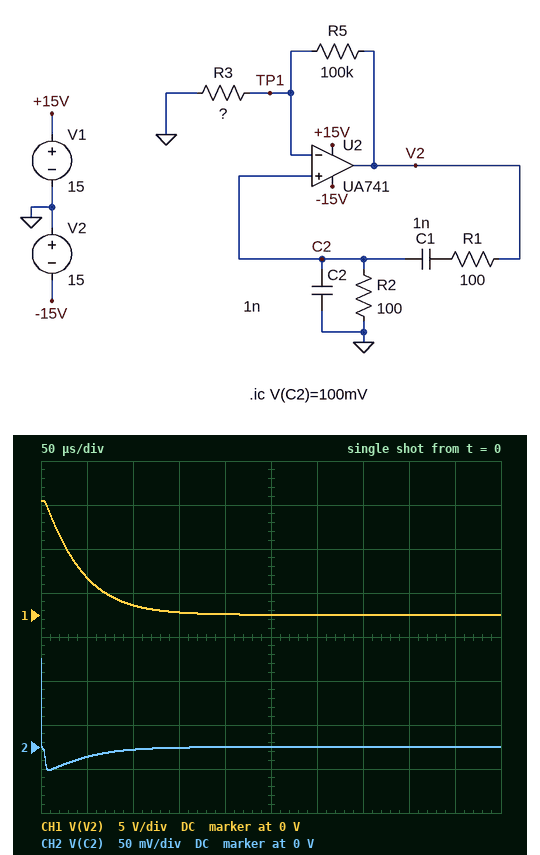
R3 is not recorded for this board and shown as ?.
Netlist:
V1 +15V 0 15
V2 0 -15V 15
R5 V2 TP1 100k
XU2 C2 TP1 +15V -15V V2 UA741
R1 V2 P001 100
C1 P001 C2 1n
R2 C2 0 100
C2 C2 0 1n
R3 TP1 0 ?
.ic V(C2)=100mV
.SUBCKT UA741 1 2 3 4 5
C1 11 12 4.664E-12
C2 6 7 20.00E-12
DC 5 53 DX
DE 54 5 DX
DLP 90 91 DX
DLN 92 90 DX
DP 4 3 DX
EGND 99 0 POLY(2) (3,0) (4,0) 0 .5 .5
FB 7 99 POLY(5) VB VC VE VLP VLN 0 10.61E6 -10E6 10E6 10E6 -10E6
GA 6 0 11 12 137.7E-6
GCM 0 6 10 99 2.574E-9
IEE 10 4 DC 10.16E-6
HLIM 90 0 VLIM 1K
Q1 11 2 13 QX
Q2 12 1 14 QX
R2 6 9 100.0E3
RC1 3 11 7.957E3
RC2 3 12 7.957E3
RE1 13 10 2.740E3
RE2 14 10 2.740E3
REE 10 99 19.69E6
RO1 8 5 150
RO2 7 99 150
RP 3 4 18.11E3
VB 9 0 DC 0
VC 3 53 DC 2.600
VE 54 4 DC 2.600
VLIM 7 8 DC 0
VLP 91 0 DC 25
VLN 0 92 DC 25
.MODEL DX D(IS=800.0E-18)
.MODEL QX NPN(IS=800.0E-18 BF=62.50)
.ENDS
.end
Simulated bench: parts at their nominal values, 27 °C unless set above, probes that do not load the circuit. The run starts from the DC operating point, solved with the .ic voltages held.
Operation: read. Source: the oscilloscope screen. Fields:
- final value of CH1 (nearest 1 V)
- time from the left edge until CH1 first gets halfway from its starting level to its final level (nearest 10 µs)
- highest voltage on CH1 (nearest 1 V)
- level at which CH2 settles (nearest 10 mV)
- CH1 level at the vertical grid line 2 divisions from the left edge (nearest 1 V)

0 V
30 µs
13 V
0 V
1 V
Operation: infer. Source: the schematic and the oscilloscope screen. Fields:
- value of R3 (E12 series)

120 Ω
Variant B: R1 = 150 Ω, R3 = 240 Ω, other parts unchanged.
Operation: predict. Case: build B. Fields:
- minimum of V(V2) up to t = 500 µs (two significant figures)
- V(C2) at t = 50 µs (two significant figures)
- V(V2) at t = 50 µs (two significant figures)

9.3 mV
-8.4 mV
1.5 V
